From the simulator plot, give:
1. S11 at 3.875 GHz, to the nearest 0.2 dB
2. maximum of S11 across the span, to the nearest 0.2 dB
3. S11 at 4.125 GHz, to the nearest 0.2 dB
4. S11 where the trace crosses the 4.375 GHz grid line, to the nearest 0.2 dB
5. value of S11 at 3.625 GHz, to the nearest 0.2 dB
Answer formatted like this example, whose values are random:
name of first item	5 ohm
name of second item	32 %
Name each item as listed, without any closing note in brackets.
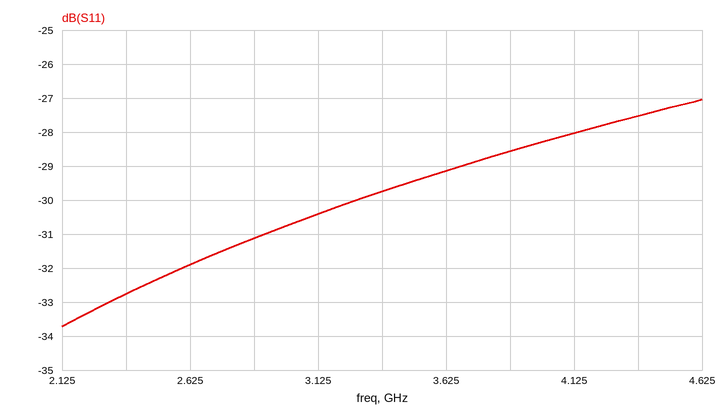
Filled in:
S11 at 3.875 GHz, to the nearest 0.2 dB	-28.6 dB
maximum of S11 across the span, to the nearest 0.2 dB	-27.0 dB
S11 at 4.125 GHz, to the nearest 0.2 dB	-28.0 dB
S11 where the trace crosses the 4.375 GHz grid line, to the nearest 0.2 dB	-27.6 dB
value of S11 at 3.625 GHz, to the nearest 0.2 dB	-29.2 dB
